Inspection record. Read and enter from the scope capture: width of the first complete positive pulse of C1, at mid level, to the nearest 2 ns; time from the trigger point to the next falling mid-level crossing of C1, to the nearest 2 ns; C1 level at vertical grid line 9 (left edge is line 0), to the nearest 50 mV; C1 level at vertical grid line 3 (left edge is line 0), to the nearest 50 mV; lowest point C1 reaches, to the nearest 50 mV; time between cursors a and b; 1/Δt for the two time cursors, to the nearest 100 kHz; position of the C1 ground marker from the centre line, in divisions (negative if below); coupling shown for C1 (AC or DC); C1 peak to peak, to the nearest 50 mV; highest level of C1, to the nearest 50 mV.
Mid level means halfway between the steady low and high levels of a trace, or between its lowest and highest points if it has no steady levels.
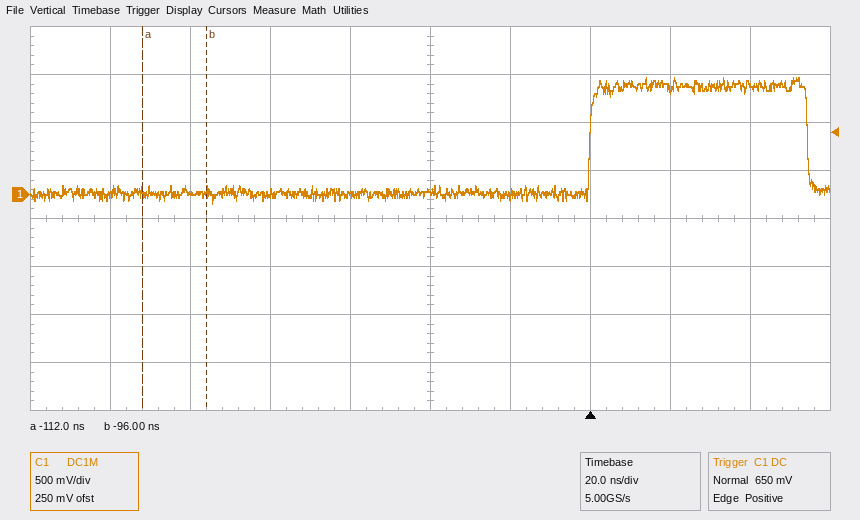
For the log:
54 ns
54 ns
1.15 V
0 mV
-100 mV
16 ns
62.5 MHz
+0.5 div
DC
1.30 V
1.20 V
